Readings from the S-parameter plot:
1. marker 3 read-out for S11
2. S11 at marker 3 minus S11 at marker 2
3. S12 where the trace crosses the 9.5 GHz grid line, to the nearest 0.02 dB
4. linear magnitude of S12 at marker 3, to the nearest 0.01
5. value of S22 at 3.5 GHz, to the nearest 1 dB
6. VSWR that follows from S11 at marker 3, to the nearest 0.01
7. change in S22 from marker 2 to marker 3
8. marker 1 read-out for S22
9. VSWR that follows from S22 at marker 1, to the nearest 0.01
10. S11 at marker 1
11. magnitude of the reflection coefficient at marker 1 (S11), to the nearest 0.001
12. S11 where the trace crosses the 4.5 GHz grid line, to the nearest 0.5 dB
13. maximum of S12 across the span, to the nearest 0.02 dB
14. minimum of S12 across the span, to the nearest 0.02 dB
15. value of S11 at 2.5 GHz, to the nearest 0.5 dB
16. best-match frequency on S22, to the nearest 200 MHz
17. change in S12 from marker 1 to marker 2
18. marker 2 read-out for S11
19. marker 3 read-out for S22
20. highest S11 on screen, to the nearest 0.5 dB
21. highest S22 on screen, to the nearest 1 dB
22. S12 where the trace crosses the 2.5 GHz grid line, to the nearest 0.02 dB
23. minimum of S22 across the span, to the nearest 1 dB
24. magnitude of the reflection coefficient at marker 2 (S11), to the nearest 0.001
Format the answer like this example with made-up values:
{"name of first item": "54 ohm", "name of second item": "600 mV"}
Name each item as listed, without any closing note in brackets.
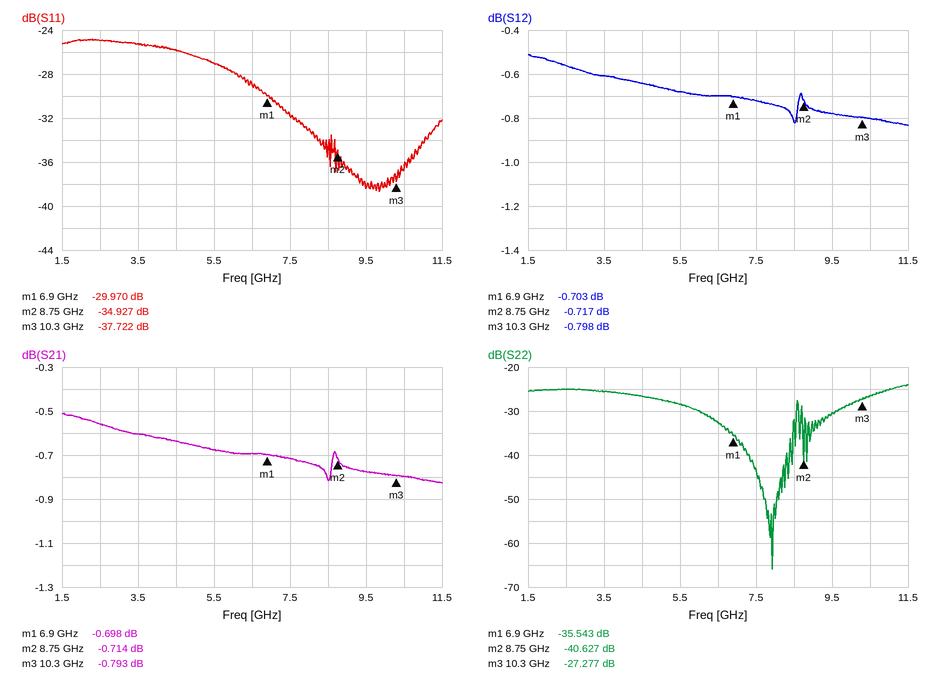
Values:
{"marker 3 read-out for S11": "-37.722 dB", "S11 at marker 3 minus S11 at marker 2": "-2.795 dB", "S12 where the trace crosses the 9.5 GHz grid line, to the nearest 0.02 dB": "-0.78 dB", "linear magnitude of S12 at marker 3, to the nearest 0.01": "0.91", "value of S22 at 3.5 GHz, to the nearest 1 dB": "-26 dB", "VSWR that follows from S11 at marker 3, to the nearest 0.01": "1.03", "change in S22 from marker 2 to marker 3": "13.350 dB", "marker 1 read-out for S22": "-35.543 dB", "VSWR that follows from S22 at marker 1, to the nearest 0.01": "1.03", "S11 at marker 1": "-29.970 dB", "magnitude of the reflection coefficient at marker 1 (S11), to the nearest 0.001": "0.032", "S11 where the trace crosses the 4.5 GHz grid line, to the nearest 0.5 dB": "-26.0 dB", "maximum of S12 across the span, to the nearest 0.02 dB": "-0.52 dB", "minimum of S12 across the span, to the nearest 0.02 dB": "-0.84 dB", "value of S11 at 2.5 GHz, to the nearest 0.5 dB": "-25.0 dB", "best-match frequency on S22, to the nearest 200 MHz": "8.0 GHz", "change in S12 from marker 1 to marker 2": "-0.014 dB", "marker 2 read-out for S11": "-34.927 dB", "marker 3 read-out for S22": "-27.277 dB", "highest S11 on screen, to the nearest 0.5 dB": "-25.0 dB", "highest S22 on screen, to the nearest 1 dB": "-24 dB", "S12 where the trace crosses the 2.5 GHz grid line, to the nearest 0.02 dB": "-0.56 dB", "minimum of S22 across the span, to the nearest 1 dB": "-66 dB", "magnitude of the reflection coefficient at marker 2 (S11), to the nearest 0.001": "0.018"}
